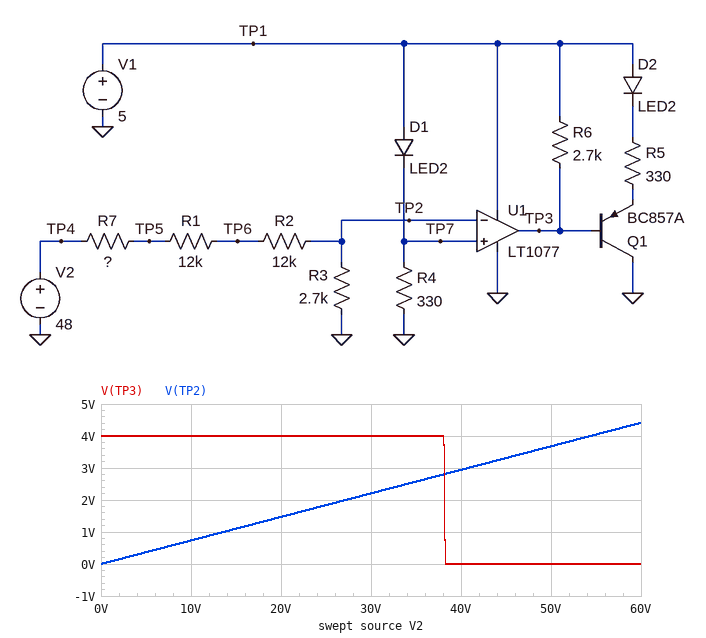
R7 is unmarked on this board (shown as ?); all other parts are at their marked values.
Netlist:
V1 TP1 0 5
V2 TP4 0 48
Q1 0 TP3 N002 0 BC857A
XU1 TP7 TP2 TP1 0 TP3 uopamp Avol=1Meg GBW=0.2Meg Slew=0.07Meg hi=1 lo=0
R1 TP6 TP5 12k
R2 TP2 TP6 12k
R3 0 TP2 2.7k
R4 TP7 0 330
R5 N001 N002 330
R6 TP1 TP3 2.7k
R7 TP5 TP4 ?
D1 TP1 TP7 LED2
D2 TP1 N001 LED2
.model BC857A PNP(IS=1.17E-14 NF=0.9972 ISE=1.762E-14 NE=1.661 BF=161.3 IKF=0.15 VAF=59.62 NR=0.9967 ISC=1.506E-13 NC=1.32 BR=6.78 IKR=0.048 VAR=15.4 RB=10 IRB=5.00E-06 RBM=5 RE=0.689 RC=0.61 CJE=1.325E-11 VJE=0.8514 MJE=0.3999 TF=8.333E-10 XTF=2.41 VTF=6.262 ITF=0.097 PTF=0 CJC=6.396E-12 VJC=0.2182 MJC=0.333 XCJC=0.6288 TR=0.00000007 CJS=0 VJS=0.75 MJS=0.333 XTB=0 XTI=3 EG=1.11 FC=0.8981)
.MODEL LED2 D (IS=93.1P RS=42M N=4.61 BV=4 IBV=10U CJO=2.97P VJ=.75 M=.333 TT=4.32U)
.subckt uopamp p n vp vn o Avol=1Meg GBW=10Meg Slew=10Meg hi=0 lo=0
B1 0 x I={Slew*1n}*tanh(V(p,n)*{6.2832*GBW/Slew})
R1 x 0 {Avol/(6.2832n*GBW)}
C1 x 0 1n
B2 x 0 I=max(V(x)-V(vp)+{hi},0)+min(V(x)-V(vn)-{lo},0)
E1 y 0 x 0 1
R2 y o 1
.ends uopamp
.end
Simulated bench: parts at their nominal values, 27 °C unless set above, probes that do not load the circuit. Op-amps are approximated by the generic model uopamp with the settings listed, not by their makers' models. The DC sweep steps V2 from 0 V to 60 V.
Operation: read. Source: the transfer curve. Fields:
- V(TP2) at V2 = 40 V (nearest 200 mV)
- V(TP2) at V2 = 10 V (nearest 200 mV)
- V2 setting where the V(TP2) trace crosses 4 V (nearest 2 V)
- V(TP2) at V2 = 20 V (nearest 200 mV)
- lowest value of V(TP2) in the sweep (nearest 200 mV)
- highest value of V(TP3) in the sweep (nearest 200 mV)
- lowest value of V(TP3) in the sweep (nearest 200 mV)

3.0 V
800 mV
54 V
1.4 V
0 V
4.0 V
0 V
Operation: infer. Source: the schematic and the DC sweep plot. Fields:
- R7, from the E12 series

10 kΩ
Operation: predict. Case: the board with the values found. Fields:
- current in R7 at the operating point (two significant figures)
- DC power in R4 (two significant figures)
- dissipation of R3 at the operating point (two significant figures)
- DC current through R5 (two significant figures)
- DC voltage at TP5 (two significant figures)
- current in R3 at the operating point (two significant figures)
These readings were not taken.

1.3 mA
24 mW
4.6 mW
6.5 mA
35 V
1.3 mA
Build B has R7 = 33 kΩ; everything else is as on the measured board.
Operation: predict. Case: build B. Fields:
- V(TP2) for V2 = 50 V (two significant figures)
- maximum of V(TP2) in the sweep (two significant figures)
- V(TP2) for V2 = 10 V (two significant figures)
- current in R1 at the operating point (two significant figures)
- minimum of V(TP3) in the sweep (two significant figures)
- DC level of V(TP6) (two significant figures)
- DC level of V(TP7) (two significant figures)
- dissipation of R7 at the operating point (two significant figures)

2.3 V
2.7 V
450 mV
800 µA
4.0 V
12 V
2.8 V
21 mW
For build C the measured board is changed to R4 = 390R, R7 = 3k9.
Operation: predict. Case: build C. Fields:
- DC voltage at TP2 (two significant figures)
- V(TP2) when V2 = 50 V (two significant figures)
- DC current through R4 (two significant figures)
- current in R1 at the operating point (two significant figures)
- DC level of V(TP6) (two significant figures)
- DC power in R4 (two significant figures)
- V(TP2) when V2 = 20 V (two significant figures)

4.2 V
4.4 V
7.3 mA
1.6 mA
23 V
21 mW
1.8 V
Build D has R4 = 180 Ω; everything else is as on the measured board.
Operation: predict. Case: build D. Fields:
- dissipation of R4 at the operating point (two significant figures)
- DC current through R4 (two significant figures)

42 mW
15 mA
